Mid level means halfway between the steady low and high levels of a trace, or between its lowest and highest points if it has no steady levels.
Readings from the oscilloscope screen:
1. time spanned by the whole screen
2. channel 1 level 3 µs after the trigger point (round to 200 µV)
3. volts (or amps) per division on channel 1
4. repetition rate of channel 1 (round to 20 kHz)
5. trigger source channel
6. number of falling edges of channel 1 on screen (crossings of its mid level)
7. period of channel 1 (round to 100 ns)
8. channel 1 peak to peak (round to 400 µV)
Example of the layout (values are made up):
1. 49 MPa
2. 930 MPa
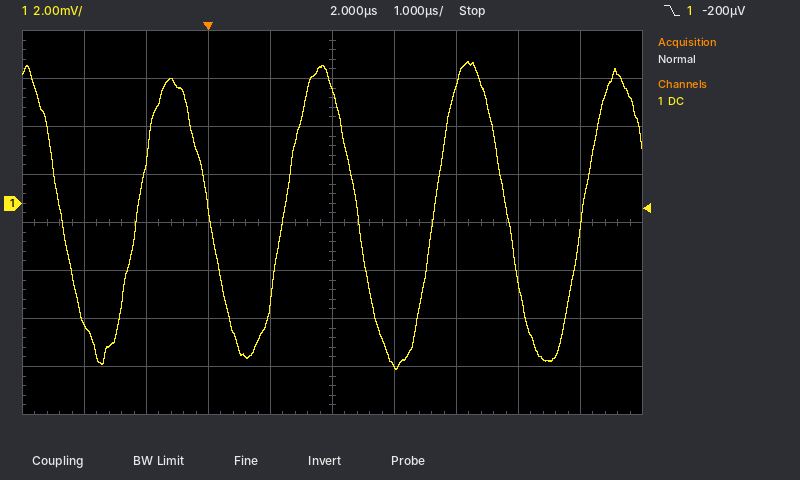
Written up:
1. 10 µs
2. -6.8 mV
3. 2 mV
4. 420 kHz
5. channel 1
6. 4
7. 2.4 µs
8. 12.8 mV
